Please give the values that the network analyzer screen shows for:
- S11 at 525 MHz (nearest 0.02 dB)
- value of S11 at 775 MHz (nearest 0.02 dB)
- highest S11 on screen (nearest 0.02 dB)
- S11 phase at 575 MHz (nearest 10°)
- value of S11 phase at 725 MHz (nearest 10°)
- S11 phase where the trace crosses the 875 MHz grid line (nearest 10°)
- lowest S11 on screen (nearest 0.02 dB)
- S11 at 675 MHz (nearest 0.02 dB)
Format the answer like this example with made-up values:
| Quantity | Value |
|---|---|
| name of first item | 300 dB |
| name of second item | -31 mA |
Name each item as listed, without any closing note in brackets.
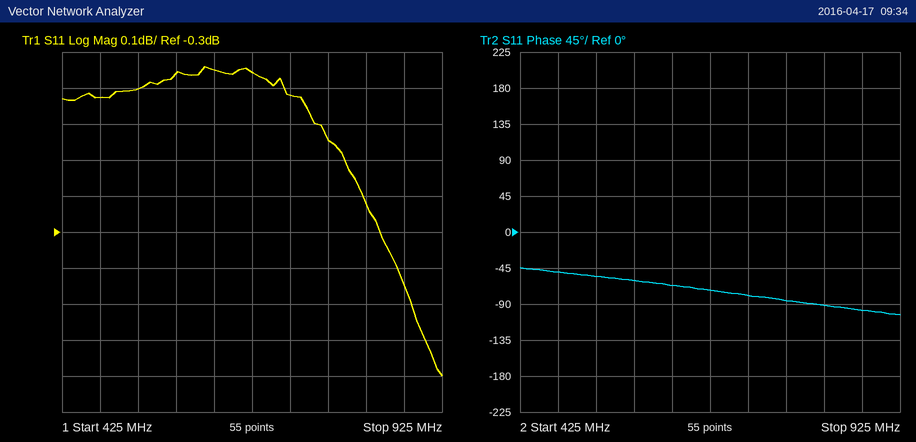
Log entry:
| Quantity | Value |
|---|---|
| S11 at 525 MHz | 0.10 dB |
| value of S11 at 775 MHz | -0.04 dB |
| highest S11 on screen | 0.16 dB |
| S11 phase at 575 MHz | -60° |
| value of S11 phase at 725 MHz | -80° |
| S11 phase where the trace crosses the 875 MHz grid line | -100° |
| lowest S11 on screen | -0.70 dB |
| S11 at 675 MHz | 0.14 dB |
